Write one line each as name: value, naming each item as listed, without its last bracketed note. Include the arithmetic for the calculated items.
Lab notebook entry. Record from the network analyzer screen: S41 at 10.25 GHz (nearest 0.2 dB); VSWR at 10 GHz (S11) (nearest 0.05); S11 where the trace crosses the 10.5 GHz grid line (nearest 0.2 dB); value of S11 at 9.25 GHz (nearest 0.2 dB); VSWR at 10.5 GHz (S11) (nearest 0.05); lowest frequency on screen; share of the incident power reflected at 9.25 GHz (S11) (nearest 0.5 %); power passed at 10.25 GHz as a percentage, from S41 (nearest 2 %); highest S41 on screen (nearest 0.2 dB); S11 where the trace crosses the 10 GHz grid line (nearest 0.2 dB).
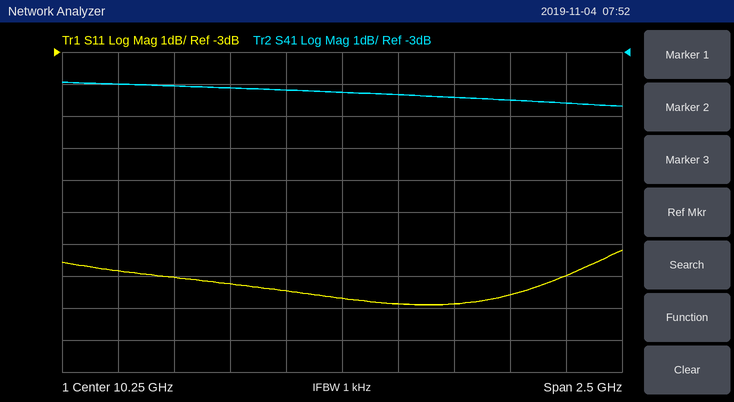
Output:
S41 at 10.25 GHz: -4.2 dB
VSWR at 10 GHz (S11): |Γ| = 10^(-10.4/20) = 0.3020; VSWR = (1 + 0.3020)/(1 − 0.3020) ≈ 1.87, so 1.85 to the nearest 0.05
S11 where the trace crosses the 10.5 GHz grid line: -10.8 dB
value of S11 at 9.25 GHz: -9.8 dB
VSWR at 10.5 GHz (S11): |Γ| = 10^(-10.8/20) = 0.2884; VSWR = (1 + 0.2884)/(1 − 0.2884) ≈ 1.81, so 1.80 to the nearest 0.05
lowest frequency on screen: 9 GHz
share of the incident power reflected at 9.25 GHz (S11): 10^(-9.8/10) ≈ 10.5 %
power passed at 10.25 GHz as a percentage, from S41: 10^(-4.2/10) ≈ 38 %
highest S41 on screen: -4.0 dB
S11 where the trace crosses the 10 GHz grid line: -10.4 dB
